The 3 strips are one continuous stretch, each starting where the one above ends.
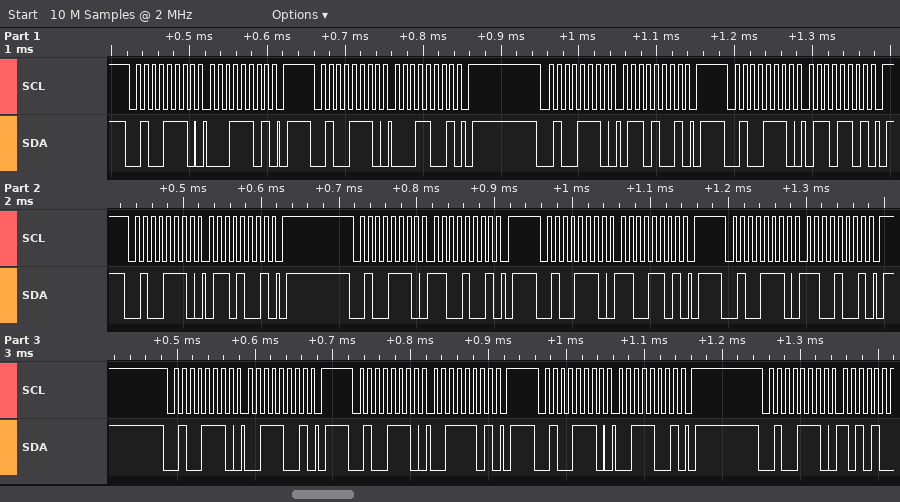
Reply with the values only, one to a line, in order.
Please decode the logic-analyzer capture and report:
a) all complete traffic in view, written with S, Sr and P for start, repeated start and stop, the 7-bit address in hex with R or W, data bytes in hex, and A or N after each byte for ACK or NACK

S 27W A 1D A P S 27W A 19 A P S 27W A 69 A P S 27W A 6D A P S 27W A 69 A P S 27W A C9 A P S 27W A CD A P S 27W A C9 A P S 27W A 39 A P S 27W A 3D A P S 27W A 39 A P S 27W A
